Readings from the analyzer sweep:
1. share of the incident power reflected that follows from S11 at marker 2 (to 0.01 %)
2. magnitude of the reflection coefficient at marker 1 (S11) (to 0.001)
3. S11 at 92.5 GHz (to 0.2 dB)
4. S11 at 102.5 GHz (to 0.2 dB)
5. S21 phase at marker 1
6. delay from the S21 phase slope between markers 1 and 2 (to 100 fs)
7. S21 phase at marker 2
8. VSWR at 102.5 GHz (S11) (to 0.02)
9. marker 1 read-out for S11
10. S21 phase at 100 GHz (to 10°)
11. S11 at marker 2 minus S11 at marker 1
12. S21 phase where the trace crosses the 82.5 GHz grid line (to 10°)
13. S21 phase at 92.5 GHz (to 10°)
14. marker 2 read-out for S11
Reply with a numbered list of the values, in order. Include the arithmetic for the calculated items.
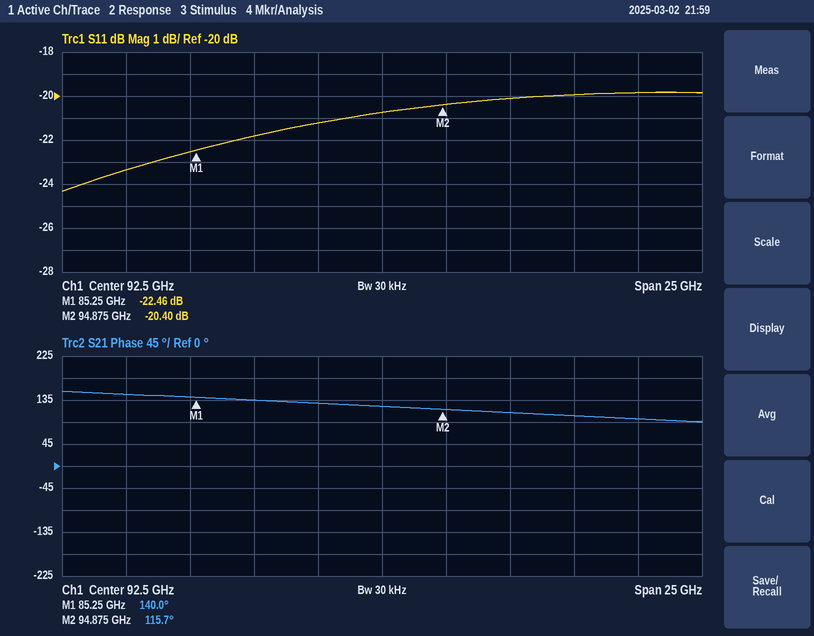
1. 10^(-20.4/10) ≈ 0.91 %
2. 10^(-22.46/20) ≈ 0.075
3. -20.8 dB
4. -19.8 dB
5. 140.0°
6. −(115.7° − (140°))/(360° × 9.625 GHz) ≈ 7.0 ps
7. 115.7°
8. |Γ| = 10^(-19.8/20) = 0.1023; VSWR = (1 + 0.1023)/(1 − 0.1023) ≈ 1.23, so 1.22 to the nearest 0.02
9. -22.46 dB
10. 100°
11. -20.4 − (-22.46) = 2.06 dB
12. 150°
13. 120°
14. -20.40 dB
